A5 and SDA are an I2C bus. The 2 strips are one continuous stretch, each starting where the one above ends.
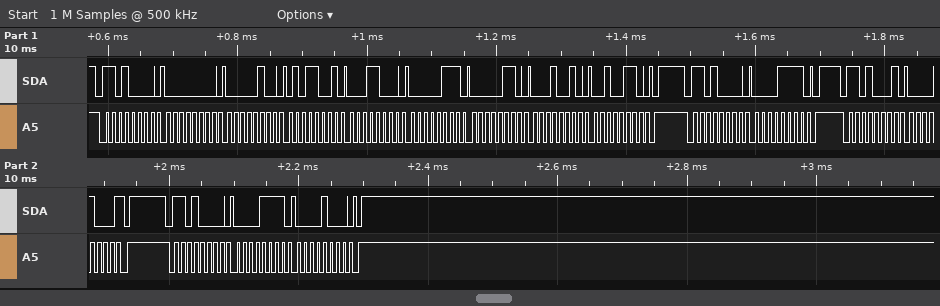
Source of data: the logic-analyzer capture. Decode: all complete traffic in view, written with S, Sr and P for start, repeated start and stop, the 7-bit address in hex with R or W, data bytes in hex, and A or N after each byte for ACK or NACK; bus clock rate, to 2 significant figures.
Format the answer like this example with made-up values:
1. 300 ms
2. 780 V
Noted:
1. S 68W A 00 A 04 A 59 A 18 A 07 A 06 A 12 A 26 A P S 68W A 0F A P S 68R A 08 N P S 68W A 0F A 08 A P
2. 100 kHz
